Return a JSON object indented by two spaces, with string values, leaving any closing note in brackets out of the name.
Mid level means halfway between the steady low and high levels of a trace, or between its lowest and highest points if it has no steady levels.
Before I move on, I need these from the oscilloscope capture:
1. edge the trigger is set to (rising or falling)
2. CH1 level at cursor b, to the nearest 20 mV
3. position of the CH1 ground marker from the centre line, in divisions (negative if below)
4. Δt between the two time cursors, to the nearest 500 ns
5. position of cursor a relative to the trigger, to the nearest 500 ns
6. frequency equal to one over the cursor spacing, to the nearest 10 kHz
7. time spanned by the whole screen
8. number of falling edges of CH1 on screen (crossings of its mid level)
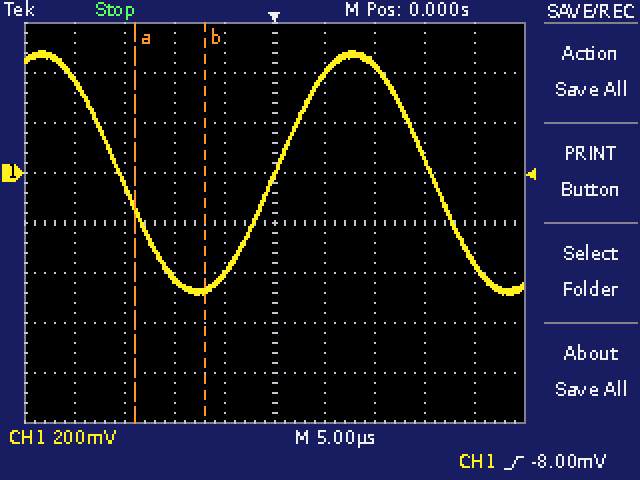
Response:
{
  "edge the trigger is set to": "rising",
  "CH1 level at cursor b, to the nearest 20 mV": "-460 mV",
  "position of the CH1 ground marker from the centre line, in divisions": "+1.0 div",
  "Δt between the two time cursors, to the nearest 500 ns": "7.0 µs",
  "position of cursor a relative to the trigger, to the nearest 500 ns": "-14.0 µs",
  "frequency equal to one over the cursor spacing, to the nearest 10 kHz": "140 kHz",
  "time spanned by the whole screen": "50 µs",
  "number of falling edges of CH1 on screen": "2"
}
